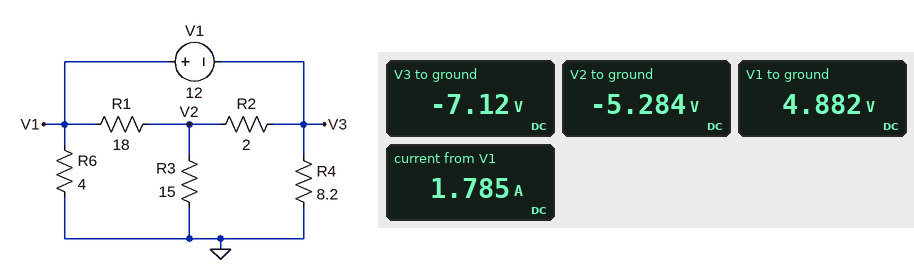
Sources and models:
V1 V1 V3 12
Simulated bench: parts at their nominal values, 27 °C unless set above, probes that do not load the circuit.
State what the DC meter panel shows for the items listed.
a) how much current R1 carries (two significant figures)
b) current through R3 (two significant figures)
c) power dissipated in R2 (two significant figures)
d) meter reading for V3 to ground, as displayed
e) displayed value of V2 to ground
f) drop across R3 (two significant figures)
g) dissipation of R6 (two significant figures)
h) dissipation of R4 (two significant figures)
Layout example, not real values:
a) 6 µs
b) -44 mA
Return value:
a) 560 mA
b) 350 mA
c) 1.7 W
d) -7.12 V
e) -5.284 V
f) 5.3 V
g) 6.0 W
h) 6.2 W
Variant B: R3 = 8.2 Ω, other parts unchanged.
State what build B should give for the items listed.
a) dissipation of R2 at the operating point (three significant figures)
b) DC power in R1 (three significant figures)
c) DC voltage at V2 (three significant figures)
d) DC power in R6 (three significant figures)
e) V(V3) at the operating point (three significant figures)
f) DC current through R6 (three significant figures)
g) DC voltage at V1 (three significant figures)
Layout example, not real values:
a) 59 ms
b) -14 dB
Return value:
a) 2.36 W
b) 5.36 W
c) -4.44 V
d) 7.26 W
e) -6.61 V
f) 1.35 A
g) 5.39 V
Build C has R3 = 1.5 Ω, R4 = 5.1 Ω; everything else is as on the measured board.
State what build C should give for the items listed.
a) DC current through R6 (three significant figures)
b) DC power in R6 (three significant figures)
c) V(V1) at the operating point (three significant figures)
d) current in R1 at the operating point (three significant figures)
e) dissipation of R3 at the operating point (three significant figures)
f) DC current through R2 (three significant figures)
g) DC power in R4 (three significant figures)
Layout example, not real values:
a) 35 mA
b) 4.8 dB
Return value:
a) 1.88 A
b) 14.1 W
c) 7.51 V
d) 500 mA
e) 1.49 W
f) 1.50 A
g) 3.95 W
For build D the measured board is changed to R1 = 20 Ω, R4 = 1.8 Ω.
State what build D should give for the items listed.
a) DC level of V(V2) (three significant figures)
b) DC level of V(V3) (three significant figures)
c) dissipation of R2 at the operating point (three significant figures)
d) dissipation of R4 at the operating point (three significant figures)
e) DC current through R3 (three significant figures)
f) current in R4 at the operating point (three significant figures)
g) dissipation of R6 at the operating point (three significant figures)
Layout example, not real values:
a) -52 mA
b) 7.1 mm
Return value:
a) -2.19 V
b) -3.54 V
c) 919 mW
d) 6.97 W
e) 146 mA
f) 1.97 A
g) 17.9 W
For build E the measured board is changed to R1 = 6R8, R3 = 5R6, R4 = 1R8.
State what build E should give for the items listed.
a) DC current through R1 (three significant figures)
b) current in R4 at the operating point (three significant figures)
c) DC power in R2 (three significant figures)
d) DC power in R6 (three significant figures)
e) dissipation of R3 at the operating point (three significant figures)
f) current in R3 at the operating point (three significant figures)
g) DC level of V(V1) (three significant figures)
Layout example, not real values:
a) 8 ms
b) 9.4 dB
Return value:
a) 1.34 A
b) 1.99 A
c) 4.24 W
d) 17.7 W
e) 79.1 mW
f) 119 mA
g) 8.42 V
